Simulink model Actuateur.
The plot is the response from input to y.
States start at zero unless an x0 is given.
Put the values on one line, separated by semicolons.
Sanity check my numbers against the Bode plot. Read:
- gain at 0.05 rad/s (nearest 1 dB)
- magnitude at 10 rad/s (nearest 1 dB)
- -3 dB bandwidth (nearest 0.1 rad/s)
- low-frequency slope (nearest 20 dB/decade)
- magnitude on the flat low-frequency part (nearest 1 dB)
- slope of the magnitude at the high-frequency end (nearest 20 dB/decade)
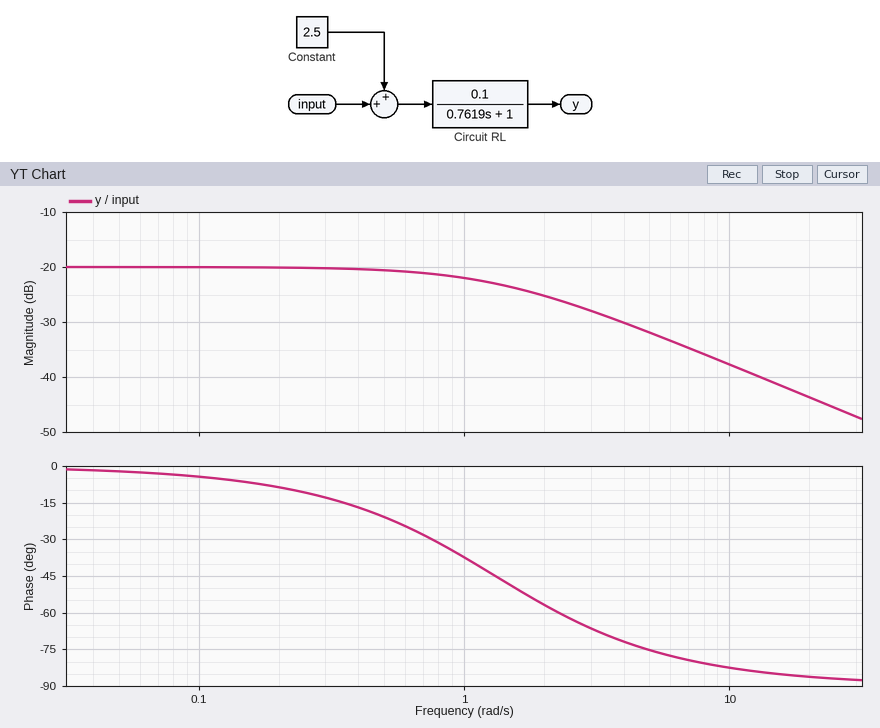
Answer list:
-20 dB; -38 dB; 1.3 rad/s; 0 dB/decade; -20 dB; -20 dB/decade
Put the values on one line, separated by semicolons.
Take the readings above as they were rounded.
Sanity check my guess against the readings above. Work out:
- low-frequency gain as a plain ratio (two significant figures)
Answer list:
0.10
